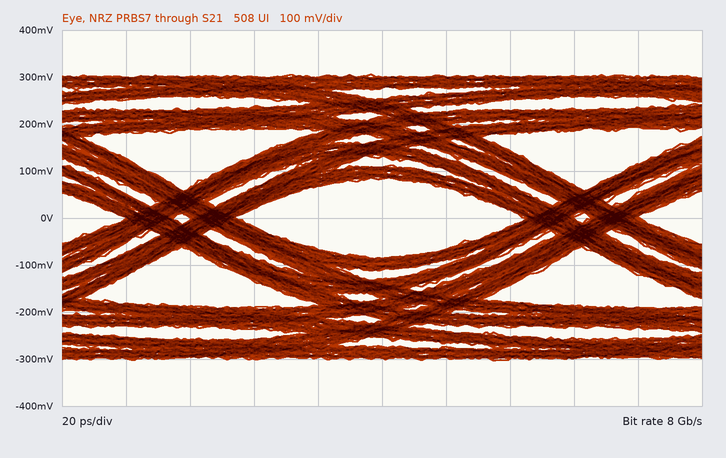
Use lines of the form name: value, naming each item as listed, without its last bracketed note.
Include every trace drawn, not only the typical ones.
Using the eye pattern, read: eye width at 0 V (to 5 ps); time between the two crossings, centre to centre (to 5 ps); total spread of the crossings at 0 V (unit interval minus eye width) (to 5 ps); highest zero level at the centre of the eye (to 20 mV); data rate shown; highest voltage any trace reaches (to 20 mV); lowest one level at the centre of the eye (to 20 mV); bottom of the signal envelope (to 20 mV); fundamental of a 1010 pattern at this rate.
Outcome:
eye width at 0 V: 90 ps
time between the two crossings, centre to centre: 125 ps
total spread of the crossings at 0 V (unit interval minus eye width): 35 ps
highest zero level at the centre of the eye: -80 mV
data rate shown: 8 Gb/s
highest voltage any trace reaches: 300 mV
lowest one level at the centre of the eye: 80 mV
bottom of the signal envelope: -300 mV
fundamental of a 1010 pattern at this rate: 4 GHz
